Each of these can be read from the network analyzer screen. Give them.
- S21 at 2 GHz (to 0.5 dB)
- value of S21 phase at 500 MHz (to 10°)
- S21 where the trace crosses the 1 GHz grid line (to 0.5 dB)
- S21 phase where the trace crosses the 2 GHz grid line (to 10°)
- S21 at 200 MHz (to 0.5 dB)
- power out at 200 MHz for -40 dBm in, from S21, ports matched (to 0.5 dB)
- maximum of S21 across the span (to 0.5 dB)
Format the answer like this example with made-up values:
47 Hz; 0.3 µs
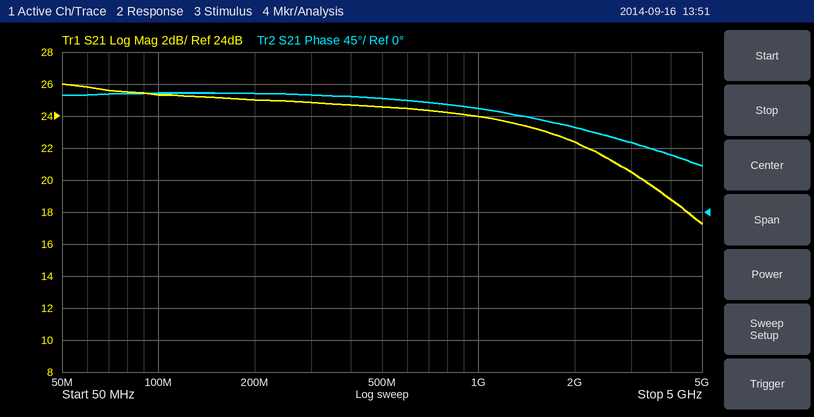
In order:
22.5 dB; 160°; 24.0 dB; 120°; 25.0 dB; -15.0 dBm; 26.0 dB
